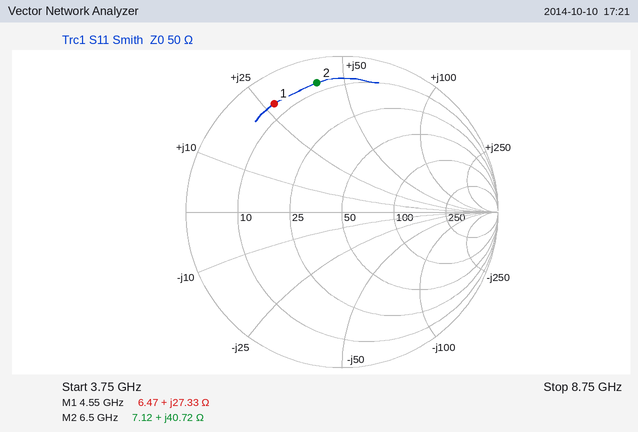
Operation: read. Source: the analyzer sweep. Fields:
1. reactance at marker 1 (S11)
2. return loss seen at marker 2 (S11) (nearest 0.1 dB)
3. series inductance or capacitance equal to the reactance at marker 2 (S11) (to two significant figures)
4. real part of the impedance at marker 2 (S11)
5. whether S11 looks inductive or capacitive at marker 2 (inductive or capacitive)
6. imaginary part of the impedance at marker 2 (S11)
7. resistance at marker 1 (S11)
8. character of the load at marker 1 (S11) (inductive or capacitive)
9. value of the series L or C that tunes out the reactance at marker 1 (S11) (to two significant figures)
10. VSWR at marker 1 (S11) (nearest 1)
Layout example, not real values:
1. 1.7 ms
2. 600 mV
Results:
1. +27.33 Ω
2. 1.5 dB
3. 1.00 nH
4. 7.12 Ω
5. inductive
6. +40.72 Ω
7. 6.47 Ω
8. inductive
9. 1.3 pF
10. 10
